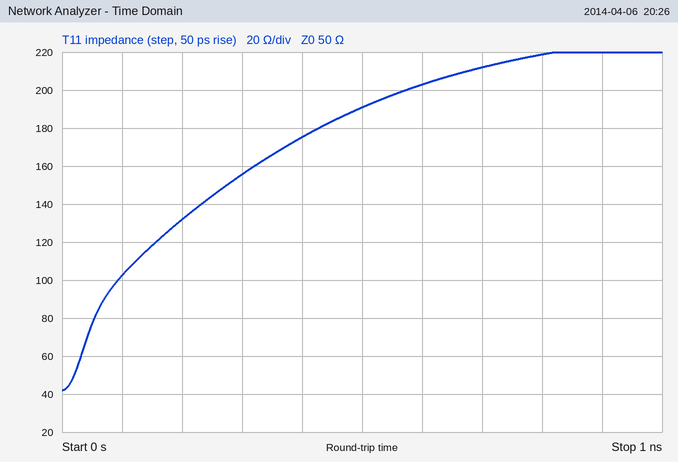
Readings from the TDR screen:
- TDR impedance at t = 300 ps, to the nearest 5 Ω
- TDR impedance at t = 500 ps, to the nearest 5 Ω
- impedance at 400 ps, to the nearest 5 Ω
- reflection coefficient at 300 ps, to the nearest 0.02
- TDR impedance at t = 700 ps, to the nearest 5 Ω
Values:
155 Ω
190 Ω
175 Ω
+0.52
210 Ω
